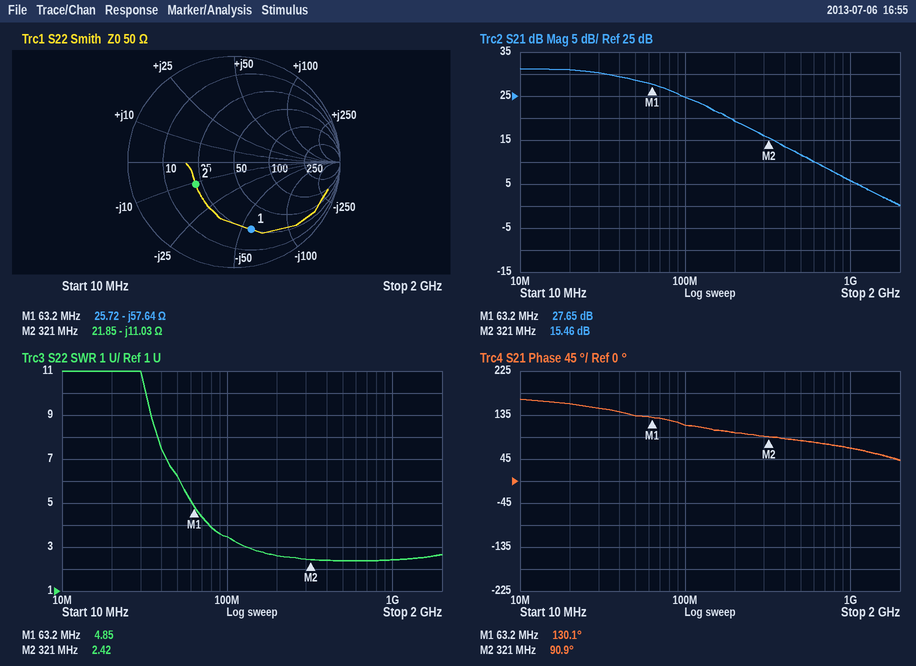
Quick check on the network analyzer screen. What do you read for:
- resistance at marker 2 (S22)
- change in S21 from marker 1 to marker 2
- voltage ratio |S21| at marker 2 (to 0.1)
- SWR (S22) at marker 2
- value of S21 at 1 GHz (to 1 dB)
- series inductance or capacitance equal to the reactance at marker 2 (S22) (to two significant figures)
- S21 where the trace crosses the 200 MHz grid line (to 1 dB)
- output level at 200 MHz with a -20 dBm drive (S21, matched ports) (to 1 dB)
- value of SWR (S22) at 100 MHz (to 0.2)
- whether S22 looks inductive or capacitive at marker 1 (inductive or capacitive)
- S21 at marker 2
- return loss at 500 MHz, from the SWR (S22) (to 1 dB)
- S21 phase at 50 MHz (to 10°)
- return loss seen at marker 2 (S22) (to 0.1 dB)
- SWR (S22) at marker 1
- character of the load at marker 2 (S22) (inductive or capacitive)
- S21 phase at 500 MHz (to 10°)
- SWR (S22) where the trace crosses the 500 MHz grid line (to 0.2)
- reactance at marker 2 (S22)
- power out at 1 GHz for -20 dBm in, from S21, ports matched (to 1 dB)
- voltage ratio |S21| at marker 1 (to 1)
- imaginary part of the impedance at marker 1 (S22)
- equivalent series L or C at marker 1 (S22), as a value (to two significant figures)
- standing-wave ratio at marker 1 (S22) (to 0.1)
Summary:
21.85 Ω
-12.19 dB
5.9
2.42
6 dB
45 pF
19 dB
-1 dBm
3.4
capacitive
15.46 dB
8 dB
130°
7.6 dB
4.85
capacitive
80°
2.4
-11.03 Ω
-14 dBm
24
-57.64 Ω
44 pF
4.8
